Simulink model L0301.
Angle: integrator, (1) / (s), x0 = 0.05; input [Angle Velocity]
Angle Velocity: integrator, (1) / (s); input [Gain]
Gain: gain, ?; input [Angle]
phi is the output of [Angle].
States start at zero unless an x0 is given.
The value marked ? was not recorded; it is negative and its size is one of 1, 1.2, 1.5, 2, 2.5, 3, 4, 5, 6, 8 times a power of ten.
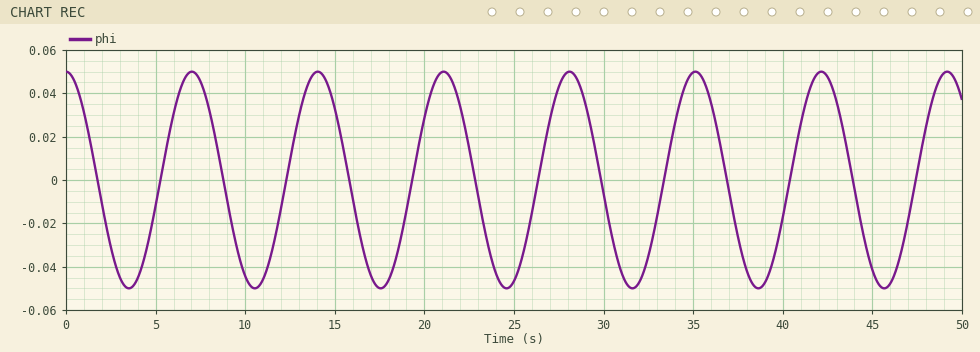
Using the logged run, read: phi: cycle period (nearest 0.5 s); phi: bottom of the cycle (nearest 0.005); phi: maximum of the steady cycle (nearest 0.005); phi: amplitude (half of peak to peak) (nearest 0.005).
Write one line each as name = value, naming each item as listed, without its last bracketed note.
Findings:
phi: cycle period = 7.0 s
phi: bottom of the cycle = -0.050
phi: maximum of the steady cycle = 0.050
phi: amplitude (half of peak to peak) = 0.050
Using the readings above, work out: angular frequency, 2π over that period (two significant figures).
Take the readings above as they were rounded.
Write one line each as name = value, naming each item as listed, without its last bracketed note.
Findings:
angular frequency, 2π over that period = 0.90 rad/s
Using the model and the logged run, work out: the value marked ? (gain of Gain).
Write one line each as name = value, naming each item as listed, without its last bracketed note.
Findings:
the value marked ? = -0.8
